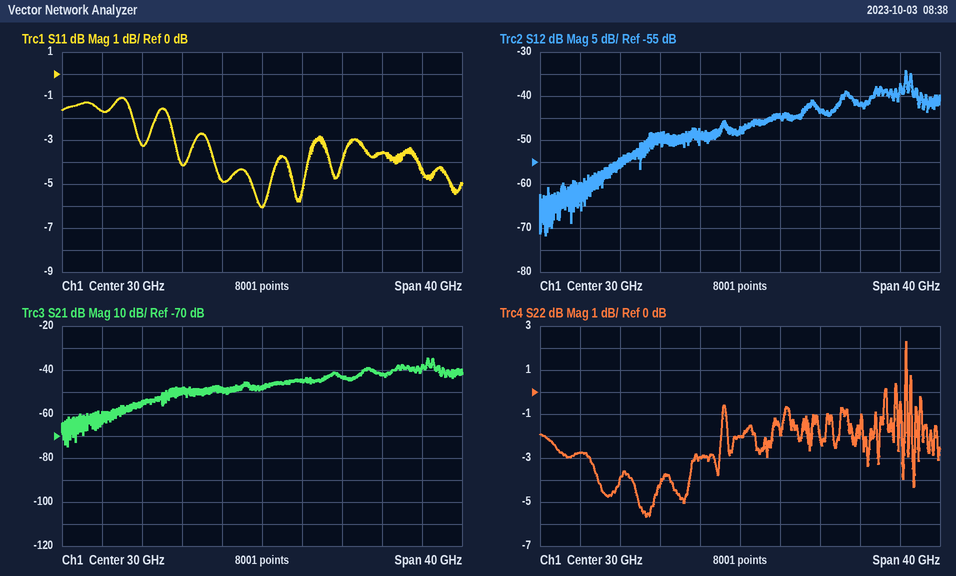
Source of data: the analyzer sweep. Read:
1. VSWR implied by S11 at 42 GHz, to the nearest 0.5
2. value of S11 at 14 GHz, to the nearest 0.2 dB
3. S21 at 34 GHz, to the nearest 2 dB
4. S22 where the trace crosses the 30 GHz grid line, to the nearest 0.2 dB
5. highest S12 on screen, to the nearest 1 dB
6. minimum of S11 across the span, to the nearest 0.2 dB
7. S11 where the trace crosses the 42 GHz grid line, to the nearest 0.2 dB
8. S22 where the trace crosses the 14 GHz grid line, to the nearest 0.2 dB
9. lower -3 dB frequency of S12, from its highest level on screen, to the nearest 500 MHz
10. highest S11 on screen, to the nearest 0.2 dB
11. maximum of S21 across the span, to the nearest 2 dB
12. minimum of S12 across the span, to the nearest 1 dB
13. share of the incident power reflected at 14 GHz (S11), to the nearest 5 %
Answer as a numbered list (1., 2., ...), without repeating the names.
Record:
1. 5.0
2. -1.6 dB
3. -44 dB
4. -2.0 dB
5. -34 dB
6. -6.0 dB
7. -3.6 dB
8. -2.8 dB
9. 46.5 GHz
10. -1.0 dB
11. -34 dB
12. -72 dB
13. 70 %
